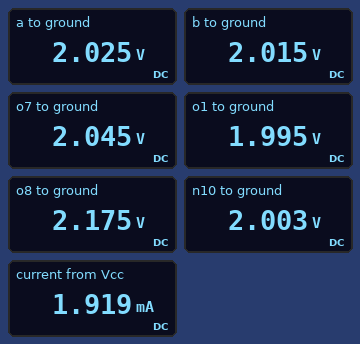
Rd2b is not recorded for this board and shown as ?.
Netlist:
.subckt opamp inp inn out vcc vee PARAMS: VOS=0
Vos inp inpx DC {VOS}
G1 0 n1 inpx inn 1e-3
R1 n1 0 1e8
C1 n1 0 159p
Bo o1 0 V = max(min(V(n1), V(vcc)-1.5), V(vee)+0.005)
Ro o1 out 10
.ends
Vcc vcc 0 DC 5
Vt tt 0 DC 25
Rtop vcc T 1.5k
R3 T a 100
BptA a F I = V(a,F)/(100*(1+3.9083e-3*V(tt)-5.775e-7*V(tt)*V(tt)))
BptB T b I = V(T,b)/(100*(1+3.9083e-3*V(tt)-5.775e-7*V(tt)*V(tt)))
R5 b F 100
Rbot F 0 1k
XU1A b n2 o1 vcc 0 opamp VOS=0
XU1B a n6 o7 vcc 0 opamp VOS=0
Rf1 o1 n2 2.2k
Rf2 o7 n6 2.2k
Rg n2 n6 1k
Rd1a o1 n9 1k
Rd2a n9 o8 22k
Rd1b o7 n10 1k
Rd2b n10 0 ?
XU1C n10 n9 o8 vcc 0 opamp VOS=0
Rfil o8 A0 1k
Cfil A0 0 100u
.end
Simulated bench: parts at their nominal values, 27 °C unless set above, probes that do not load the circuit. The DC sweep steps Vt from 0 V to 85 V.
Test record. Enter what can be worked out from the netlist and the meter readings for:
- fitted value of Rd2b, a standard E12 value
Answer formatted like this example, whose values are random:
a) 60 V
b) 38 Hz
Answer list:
a) 47 kΩ
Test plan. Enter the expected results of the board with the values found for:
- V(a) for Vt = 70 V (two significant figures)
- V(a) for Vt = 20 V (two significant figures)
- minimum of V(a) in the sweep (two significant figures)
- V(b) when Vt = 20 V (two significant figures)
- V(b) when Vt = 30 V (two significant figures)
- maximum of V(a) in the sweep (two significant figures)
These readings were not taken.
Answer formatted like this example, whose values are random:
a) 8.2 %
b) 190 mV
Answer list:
a) 2.0 V
b) 2.0 V
c) 2.0 V
d) 2.0 V
e) 2.0 V
f) 2.0 V
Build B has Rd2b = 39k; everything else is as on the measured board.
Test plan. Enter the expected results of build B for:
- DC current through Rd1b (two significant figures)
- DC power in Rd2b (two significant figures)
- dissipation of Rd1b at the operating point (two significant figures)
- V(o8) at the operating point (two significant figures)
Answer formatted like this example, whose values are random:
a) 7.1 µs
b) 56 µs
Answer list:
a) 51 µA
b) 100 µW
c) 2.6 µW
d) 2.0 V
